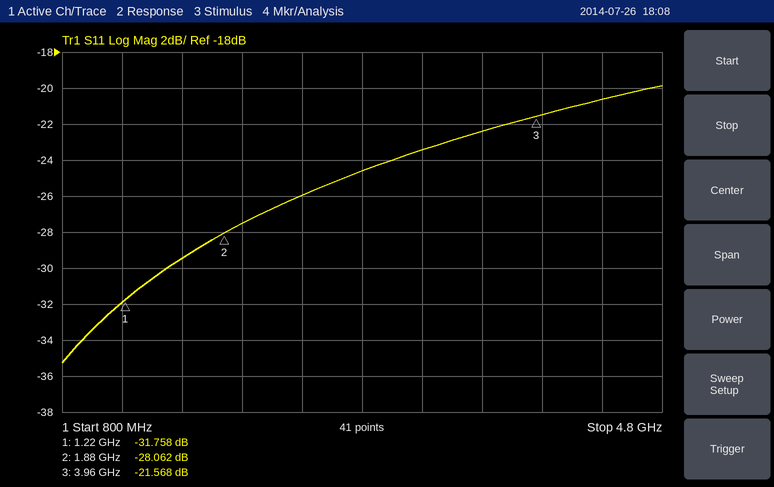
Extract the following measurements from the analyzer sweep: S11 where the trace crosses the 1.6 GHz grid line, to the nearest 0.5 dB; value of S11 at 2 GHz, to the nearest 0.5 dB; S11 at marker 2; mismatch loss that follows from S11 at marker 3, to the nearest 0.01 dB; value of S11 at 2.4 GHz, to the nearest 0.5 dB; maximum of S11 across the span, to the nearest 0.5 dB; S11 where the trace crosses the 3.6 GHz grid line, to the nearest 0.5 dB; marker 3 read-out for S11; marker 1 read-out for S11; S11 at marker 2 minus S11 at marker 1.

-29.5 dB
-27.5 dB
-28.062 dB
0.03 dB
-26.0 dB
-20.0 dB
-22.5 dB
-21.568 dB
-31.758 dB
3.696 dB
